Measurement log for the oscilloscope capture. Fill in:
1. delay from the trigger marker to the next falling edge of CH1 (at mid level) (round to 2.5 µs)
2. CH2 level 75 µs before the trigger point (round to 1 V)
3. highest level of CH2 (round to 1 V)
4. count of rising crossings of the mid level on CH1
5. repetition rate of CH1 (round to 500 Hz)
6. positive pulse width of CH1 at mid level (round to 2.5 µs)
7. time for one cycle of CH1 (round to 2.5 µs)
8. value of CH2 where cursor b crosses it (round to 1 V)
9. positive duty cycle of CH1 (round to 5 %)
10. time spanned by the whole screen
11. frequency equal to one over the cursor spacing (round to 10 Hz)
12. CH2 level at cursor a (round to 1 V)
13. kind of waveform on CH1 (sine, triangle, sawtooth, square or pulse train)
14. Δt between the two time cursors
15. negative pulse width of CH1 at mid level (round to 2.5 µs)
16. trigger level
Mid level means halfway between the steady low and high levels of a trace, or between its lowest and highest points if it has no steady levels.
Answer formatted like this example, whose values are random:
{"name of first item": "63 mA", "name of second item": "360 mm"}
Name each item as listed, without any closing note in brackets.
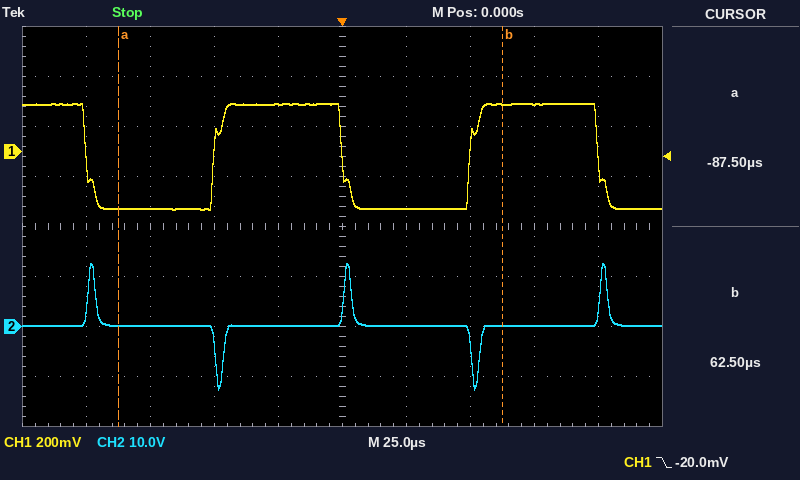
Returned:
{"delay from the trigger marker to the next falling edge of CH1 (at mid level)": "100.0 µs", "CH2 level 75 µs before the trigger point": "0 V", "highest level of CH2": "13 V", "count of rising crossings of the mid level on CH1": "2", "repetition rate of CH1": "10.0 kHz", "positive pulse width of CH1 at mid level": "50.0 µs", "time for one cycle of CH1": "100.0 µs", "value of CH2 where cursor b crosses it": "0 V", "positive duty cycle of CH1": "50 %", "time spanned by the whole screen": "250 µs", "frequency equal to one over the cursor spacing": "6.67 kHz", "CH2 level at cursor a": "0 V", "kind of waveform on CH1": "square", "Δt between the two time cursors": "150.0 µs", "negative pulse width of CH1 at mid level": "50.0 µs", "trigger level": "-20.0 mV"}
